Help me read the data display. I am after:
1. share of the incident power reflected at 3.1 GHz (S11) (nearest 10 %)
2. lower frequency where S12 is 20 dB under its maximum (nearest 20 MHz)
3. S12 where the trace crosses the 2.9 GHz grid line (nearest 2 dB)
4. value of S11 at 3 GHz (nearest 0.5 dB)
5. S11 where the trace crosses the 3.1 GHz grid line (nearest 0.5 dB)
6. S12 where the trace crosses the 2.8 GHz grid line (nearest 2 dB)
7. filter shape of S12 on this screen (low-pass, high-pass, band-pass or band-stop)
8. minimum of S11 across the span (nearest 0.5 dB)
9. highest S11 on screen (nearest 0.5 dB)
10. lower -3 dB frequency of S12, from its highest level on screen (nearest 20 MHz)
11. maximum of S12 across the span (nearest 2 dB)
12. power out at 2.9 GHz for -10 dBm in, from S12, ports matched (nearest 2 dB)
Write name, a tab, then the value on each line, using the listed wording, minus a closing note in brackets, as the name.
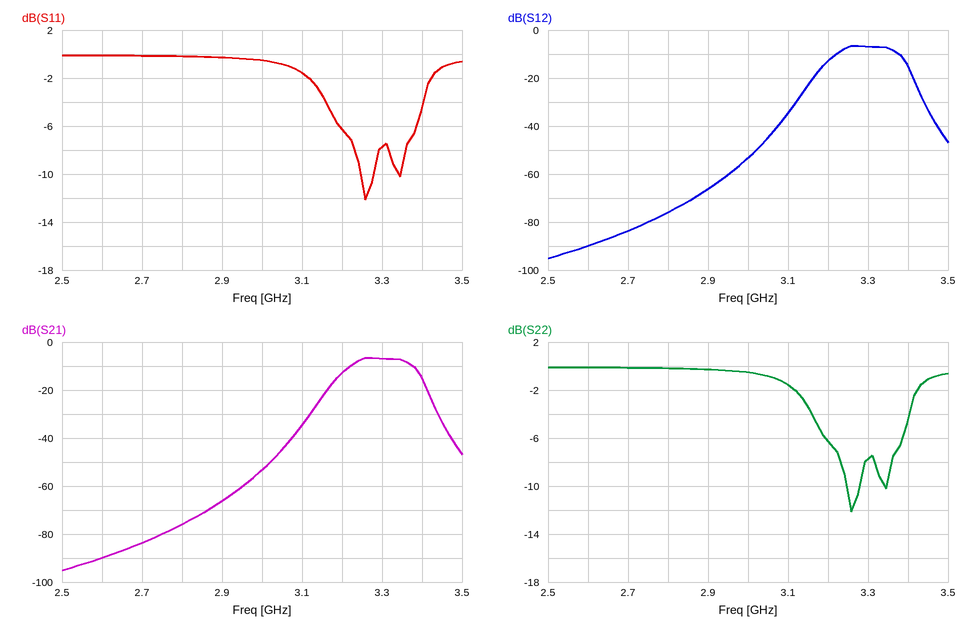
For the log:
share of the incident power reflected at 3.1 GHz (S11)	70 %
lower frequency where S12 is 20 dB under its maximum	3.14 GHz
S12 where the trace crosses the 2.9 GHz grid line	-66 dB
value of S11 at 3 GHz	-0.5 dB
S11 where the trace crosses the 3.1 GHz grid line	-1.5 dB
S12 where the trace crosses the 2.8 GHz grid line	-76 dB
filter shape of S12 on this screen	band-pass
minimum of S11 across the span	-12.0 dB
highest S11 on screen	0.0 dB
lower -3 dB frequency of S12, from its highest level on screen	3.22 GHz
maximum of S12 across the span	-6 dB
power out at 2.9 GHz for -10 dBm in, from S12, ports matched	-76 dBm
